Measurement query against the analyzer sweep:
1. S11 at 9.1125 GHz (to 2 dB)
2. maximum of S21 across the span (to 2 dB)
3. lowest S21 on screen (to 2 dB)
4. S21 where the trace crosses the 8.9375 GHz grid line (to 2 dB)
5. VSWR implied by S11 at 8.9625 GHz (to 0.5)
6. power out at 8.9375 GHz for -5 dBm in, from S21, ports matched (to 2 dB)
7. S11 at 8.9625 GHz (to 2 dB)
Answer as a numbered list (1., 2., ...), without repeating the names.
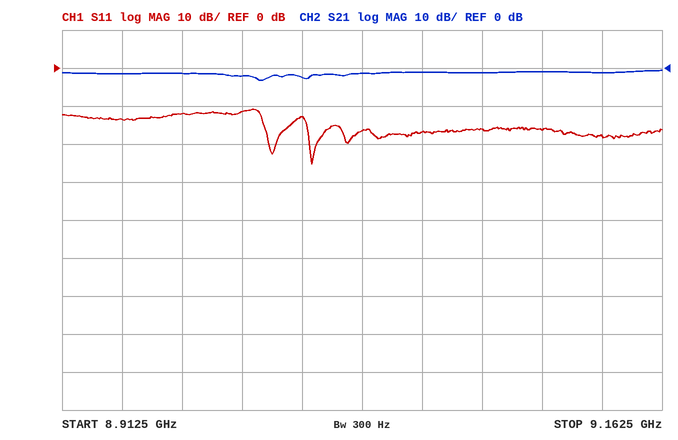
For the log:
1. -16 dB
2. 0 dB
3. -4 dB
4. -2 dB
5. 1.5
6. -6 dBm
7. -12 dB
